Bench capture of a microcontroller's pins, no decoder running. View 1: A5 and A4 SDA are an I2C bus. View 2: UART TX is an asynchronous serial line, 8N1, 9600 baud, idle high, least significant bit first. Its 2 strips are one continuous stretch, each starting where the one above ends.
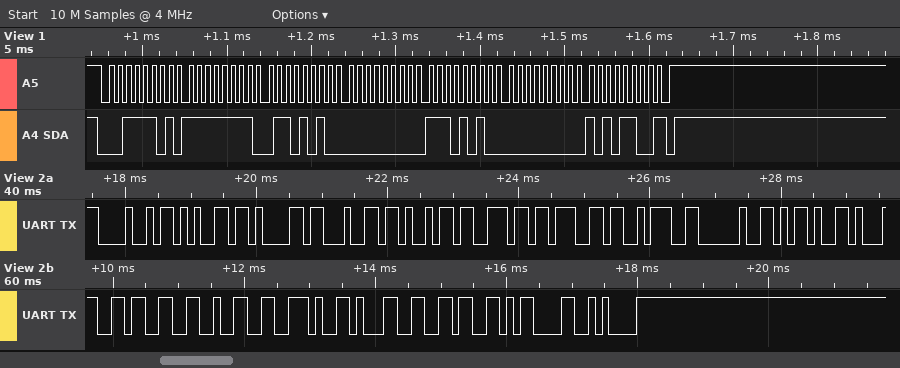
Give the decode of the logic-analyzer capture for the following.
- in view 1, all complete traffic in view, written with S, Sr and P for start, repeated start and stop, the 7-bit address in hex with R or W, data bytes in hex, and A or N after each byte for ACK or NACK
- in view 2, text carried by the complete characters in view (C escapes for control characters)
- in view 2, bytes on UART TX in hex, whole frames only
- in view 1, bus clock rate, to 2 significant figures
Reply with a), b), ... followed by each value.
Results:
a) S 1ER A FF A 6A A 00 A EA A 00 A AC N P
b) "Heading: -132.16\r\n"
c) 0x48 0x65 0x61 0x64 0x69 0x6E 0x67 0x3A 0x20 0x2D 0x31 0x33 0x32 0x2E 0x31 0x36 0x0D 0x0A
d) 100 kHz
